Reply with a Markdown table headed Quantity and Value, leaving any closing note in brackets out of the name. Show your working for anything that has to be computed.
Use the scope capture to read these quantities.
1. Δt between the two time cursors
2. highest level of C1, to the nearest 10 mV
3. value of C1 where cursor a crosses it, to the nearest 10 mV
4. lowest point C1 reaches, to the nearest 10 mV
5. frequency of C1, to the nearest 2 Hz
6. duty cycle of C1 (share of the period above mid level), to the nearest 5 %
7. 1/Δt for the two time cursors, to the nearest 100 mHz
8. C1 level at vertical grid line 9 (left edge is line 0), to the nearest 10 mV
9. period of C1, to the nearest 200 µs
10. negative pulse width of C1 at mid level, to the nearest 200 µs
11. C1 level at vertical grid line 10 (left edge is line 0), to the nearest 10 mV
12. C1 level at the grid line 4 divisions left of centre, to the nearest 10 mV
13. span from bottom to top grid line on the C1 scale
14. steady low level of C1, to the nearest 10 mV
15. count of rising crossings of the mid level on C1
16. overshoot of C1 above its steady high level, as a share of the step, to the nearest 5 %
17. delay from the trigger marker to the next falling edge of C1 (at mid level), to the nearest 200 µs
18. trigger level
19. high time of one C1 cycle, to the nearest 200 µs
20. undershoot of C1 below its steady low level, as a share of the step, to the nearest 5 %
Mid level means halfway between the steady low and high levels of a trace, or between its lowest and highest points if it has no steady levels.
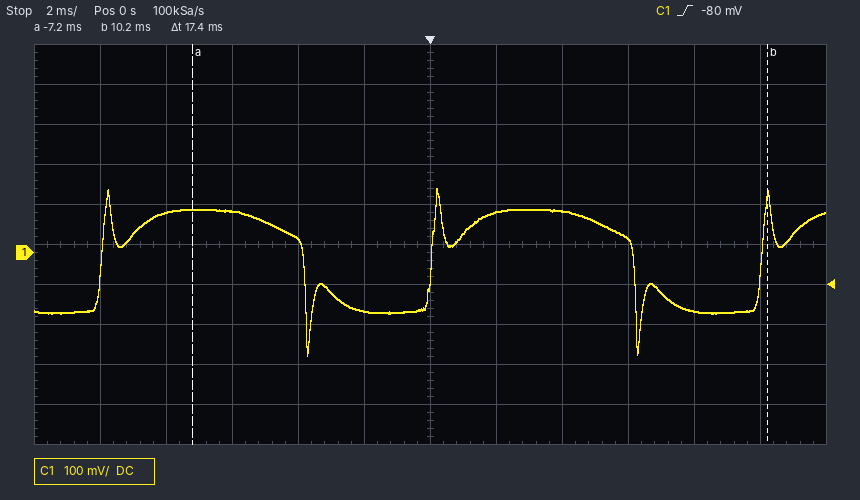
| Quantity | Value |
|---|---|
| Δt between the two time cursors | 17.4 ms |
| highest level of C1, to the nearest 10 mV | 160 mV |
| value of C1 where cursor a crosses it, to the nearest 10 mV | 110 mV |
| lowest point C1 reaches, to the nearest 10 mV | -260 mV |
| frequency of C1, to the nearest 2 Hz | 1 / 10.0 ms ≈ 100 Hz |
| duty cycle of C1 (share of the period above mid level), to the nearest 5 % | 6.2 ms / 10.0 ms ≈ 62.0 %, so 60 % to the nearest 5 % |
| 1/Δt for the two time cursors, to the nearest 100 mHz | 1 / 17.4 ms ≈ 57.5 Hz |
| C1 level at vertical grid line 9 (left edge is line 0), to the nearest 10 mV | 30 mV |
| period of C1, to the nearest 200 µs | 10.0 ms |
| negative pulse width of C1 at mid level, to the nearest 200 µs | 3.8 ms |
| C1 level at vertical grid line 10 (left edge is line 0), to the nearest 10 mV | -150 mV |
| C1 level at the grid line 4 divisions left of centre, to the nearest 10 mV | 100 mV |
| span from bottom to top grid line on the C1 scale | 1 V |
| steady low level of C1, to the nearest 10 mV | -150 mV |
| count of rising crossings of the mid level on C1 | 3 |
| overshoot of C1 above its steady high level, as a share of the step, to the nearest 5 % | 20 % |
| delay from the trigger marker to the next falling edge of C1 (at mid level), to the nearest 200 µs | 6.2 ms |
| trigger level | -80 mV |
| high time of one C1 cycle, to the nearest 200 µs | 6.2 ms |
| undershoot of C1 below its steady low level, as a share of the step, to the nearest 5 % | 40 % |
